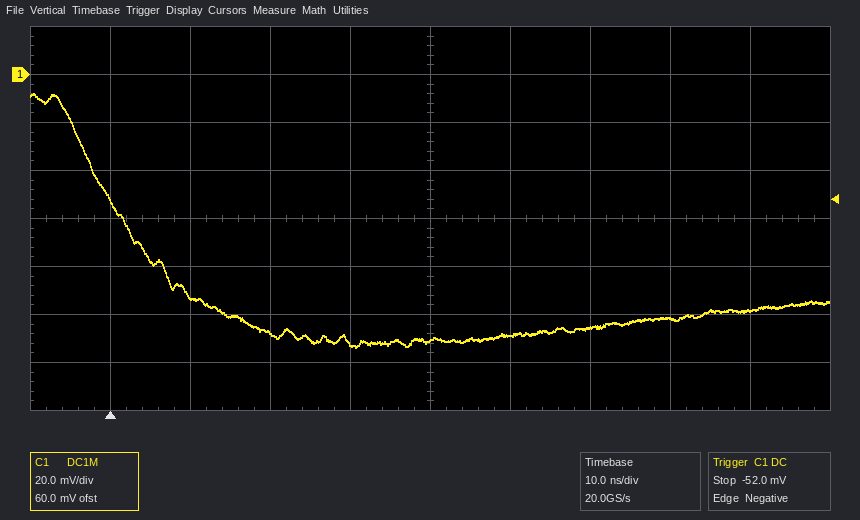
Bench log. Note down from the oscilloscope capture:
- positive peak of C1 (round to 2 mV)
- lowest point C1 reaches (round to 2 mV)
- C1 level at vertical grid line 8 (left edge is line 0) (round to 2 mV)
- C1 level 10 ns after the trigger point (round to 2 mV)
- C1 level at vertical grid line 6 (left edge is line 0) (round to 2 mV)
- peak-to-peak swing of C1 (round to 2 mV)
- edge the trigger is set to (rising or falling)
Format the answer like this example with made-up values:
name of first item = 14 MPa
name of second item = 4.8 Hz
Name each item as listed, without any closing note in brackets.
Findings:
positive peak of C1 = -8 mV
lowest point C1 reaches = -114 mV
C1 level at vertical grid line 8 (left edge is line 0) = -102 mV
C1 level 10 ns after the trigger point = -92 mV
C1 level at vertical grid line 6 (left edge is line 0) = -108 mV
peak-to-peak swing of C1 = 106 mV
edge the trigger is set to = falling
